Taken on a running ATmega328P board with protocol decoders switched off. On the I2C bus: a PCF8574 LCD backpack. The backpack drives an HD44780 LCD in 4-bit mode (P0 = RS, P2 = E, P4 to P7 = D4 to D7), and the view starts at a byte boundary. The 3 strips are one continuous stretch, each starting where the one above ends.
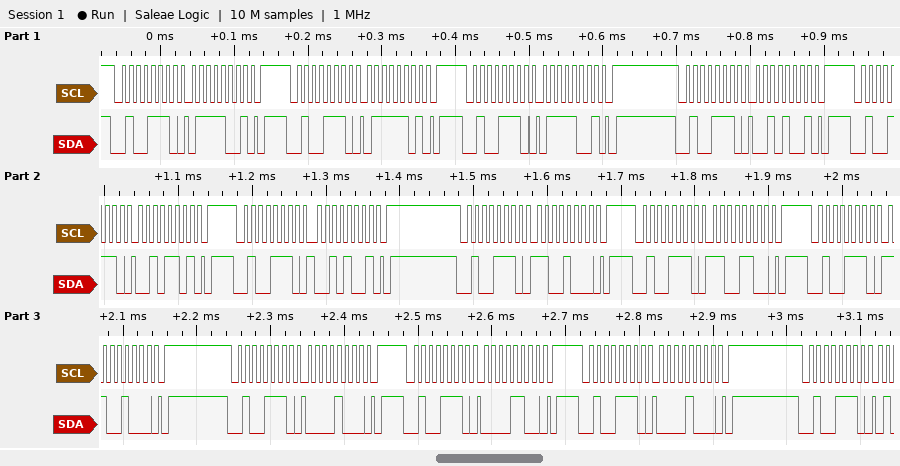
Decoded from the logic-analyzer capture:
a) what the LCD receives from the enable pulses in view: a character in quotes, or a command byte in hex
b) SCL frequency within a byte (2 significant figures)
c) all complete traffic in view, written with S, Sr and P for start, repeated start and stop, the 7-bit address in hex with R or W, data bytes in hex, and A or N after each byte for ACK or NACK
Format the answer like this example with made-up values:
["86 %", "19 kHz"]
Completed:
["'r' 0xC0", "100 kHz", "S 27W A 79 A P S 27W A 7D A P S 27W A 79 A P S 27W A 29 A P S 27W A 2D A P S 27W A 29 A P S 27W A C8 A P S 27W A CC A P S 27W A C8 A P S 27W A 08 A P S 27W A 0C A P S 27W A 08 A P S 27W A"]
